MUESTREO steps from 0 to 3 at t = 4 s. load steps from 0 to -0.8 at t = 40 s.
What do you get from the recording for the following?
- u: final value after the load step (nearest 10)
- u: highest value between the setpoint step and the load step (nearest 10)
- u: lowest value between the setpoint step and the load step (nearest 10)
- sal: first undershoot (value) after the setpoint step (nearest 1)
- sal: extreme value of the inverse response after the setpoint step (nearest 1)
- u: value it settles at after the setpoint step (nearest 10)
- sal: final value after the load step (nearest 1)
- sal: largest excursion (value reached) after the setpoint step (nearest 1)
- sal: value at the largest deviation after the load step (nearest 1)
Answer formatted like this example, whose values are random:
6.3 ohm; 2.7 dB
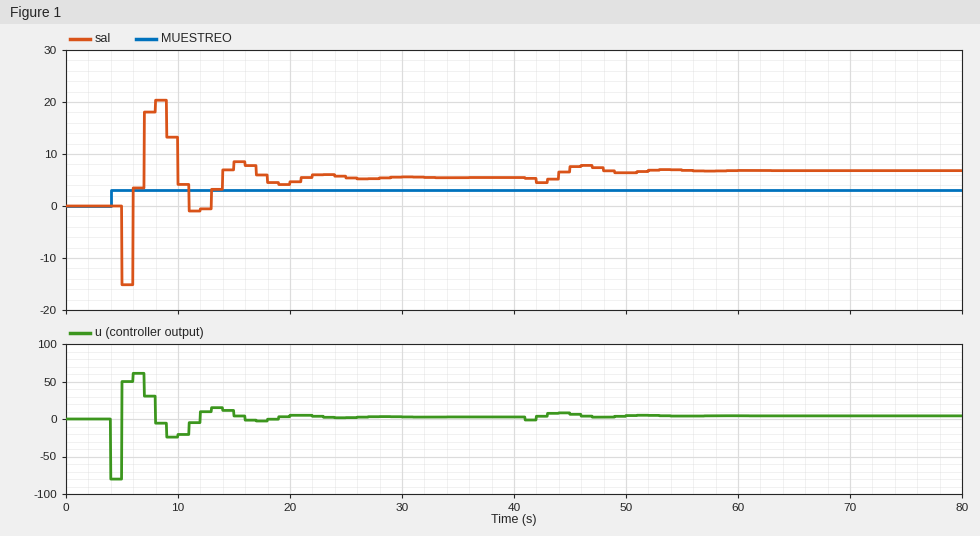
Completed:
0; 60; -80; -1; -15; 0; 7; 20; 8
